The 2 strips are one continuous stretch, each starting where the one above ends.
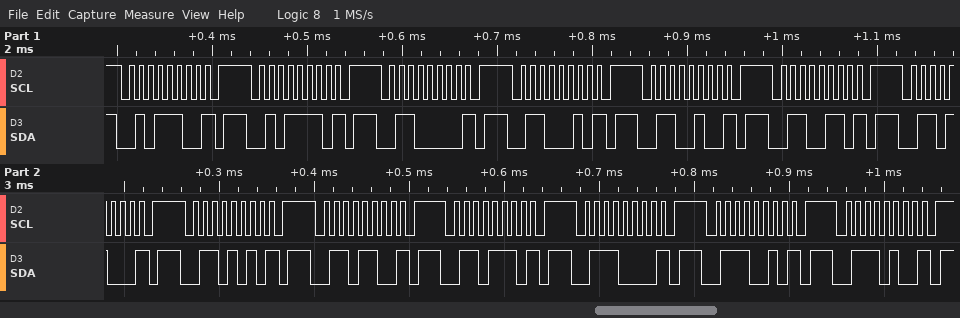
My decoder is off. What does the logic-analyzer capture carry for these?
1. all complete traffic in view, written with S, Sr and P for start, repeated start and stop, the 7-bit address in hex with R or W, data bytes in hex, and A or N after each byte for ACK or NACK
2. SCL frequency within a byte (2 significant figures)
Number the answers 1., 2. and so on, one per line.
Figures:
1. S 2EW N P S 2FW N P S 30W N P S 31W N P S 32W N P S 33W N P S 34W N P S 35W N P S 36W N P S 37W N P S 38W N P S 39W N P S 3AW N P
2. 100 kHz
